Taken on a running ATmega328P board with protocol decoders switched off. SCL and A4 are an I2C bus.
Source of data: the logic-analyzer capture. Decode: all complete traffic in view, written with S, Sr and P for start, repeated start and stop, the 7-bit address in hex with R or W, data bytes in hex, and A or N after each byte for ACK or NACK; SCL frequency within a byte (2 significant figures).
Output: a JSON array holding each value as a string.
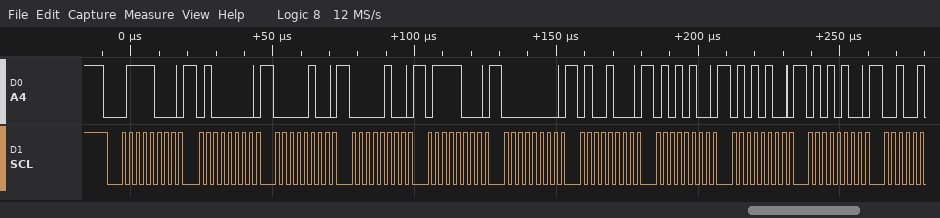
["S 3CW A 40 A 04 A 04 A 78 A 00 A 48 A 54 A 54 A 54 A", "400 kHz"]
